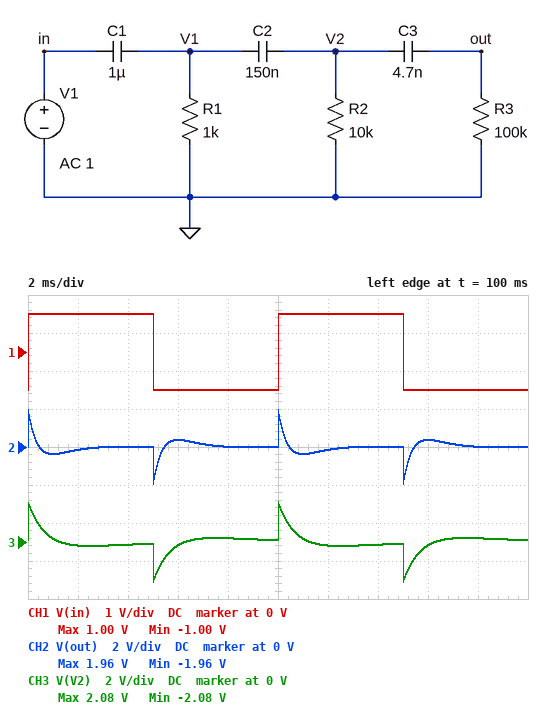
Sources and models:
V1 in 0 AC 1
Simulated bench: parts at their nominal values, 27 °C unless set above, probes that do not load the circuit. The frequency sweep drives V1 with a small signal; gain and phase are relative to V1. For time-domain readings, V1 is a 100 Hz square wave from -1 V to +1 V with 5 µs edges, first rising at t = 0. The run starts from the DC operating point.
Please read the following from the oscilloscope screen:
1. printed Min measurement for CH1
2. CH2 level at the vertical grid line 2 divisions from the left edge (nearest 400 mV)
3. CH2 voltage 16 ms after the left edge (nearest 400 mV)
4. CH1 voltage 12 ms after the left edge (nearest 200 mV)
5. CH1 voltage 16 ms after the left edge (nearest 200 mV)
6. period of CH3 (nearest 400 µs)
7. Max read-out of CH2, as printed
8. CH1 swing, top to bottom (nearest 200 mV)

-1.00 V
0 V
400 mV
1.0 V
-1.0 V
10.0 ms
1.96 V
2.0 V
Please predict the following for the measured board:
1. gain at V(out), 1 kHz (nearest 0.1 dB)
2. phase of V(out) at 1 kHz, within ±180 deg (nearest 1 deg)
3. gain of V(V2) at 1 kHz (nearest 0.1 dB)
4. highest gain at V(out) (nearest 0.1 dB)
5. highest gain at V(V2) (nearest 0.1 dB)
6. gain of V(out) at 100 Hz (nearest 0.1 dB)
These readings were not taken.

-0.7 dB
35 deg
-0.2 dB
0 dB
0 dB
-20.3 dB
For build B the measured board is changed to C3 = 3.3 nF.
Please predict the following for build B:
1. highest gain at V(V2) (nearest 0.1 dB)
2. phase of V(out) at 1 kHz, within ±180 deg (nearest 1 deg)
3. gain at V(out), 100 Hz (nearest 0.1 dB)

0 dB
42 deg
-23.2 dB
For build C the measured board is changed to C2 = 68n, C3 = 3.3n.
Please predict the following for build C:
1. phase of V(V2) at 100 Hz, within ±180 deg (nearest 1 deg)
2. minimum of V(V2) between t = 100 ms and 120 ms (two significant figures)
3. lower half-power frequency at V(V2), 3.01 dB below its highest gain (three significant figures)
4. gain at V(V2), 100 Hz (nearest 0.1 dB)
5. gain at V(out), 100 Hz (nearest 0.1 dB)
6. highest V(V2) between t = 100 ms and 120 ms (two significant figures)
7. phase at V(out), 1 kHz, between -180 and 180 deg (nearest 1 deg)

123 deg
-2.0 V
346 Hz
-13.9 dB
-27.8 dB
2.0 V
50 deg
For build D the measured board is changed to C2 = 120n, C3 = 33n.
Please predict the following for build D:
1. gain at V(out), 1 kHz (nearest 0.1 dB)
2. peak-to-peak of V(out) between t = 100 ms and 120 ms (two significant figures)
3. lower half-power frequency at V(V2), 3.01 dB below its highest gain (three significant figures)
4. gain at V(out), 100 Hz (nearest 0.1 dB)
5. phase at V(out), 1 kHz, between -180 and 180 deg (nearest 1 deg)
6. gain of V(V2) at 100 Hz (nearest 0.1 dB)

-0.3 dB
4.0 V
259 Hz
-11.8 dB
21 deg
-10.9 dB
